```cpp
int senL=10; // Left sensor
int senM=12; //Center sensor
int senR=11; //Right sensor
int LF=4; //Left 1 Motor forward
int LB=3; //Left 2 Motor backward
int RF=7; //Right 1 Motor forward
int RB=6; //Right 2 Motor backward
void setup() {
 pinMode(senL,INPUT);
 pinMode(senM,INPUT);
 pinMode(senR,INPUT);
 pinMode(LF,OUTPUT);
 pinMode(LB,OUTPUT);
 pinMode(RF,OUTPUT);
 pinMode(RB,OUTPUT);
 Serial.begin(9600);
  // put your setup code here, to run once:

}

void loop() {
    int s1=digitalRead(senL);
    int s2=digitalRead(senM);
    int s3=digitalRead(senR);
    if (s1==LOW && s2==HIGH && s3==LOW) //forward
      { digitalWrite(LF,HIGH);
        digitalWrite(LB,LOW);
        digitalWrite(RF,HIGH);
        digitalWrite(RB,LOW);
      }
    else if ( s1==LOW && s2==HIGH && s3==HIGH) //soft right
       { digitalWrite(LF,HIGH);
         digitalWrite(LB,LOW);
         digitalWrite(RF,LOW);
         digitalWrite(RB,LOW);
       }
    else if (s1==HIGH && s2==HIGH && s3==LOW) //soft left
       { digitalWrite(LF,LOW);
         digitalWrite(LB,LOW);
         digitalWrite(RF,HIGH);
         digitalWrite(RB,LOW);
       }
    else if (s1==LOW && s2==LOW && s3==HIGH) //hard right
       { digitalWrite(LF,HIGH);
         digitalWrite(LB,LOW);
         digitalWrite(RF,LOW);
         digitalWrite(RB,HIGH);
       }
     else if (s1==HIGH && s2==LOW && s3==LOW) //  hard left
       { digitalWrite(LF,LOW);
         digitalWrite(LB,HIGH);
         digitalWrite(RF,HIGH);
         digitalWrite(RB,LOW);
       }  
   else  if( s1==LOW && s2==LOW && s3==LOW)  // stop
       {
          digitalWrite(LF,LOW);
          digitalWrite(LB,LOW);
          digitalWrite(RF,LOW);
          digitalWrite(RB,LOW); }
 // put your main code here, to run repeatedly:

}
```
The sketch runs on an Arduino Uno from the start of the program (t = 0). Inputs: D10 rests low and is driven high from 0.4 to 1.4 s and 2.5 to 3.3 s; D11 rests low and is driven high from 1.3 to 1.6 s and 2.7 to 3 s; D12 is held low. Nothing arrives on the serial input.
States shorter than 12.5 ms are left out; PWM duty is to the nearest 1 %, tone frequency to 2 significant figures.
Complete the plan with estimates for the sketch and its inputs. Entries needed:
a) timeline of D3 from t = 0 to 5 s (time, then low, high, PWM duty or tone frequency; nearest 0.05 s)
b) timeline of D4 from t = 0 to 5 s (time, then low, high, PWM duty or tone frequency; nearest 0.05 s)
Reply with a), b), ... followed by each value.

a) 0 s low; 0.4 s high; 1.4 s low; 2.5 s high; 3.3 s low
b) 0 s low; 1.4 s high; 1.6 s low
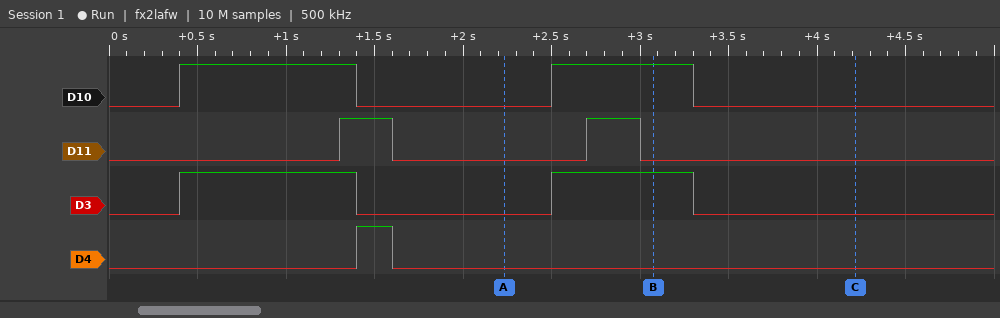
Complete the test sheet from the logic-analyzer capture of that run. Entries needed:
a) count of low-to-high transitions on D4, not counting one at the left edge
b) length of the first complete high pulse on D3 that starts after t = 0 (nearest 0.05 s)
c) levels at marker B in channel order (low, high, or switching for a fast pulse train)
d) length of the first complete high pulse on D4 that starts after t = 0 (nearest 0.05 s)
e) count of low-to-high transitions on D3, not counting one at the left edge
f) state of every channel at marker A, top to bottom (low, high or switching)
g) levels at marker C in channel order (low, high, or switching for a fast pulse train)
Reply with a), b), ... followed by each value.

a) 1
b) 1.00 s
c) D10 high, D11 low, D3 high, D4 low
d) 0.20 s
e) 2
f) D10 low, D11 low, D3 low, D4 low
g) D10 low, D11 low, D3 low, D4 low
